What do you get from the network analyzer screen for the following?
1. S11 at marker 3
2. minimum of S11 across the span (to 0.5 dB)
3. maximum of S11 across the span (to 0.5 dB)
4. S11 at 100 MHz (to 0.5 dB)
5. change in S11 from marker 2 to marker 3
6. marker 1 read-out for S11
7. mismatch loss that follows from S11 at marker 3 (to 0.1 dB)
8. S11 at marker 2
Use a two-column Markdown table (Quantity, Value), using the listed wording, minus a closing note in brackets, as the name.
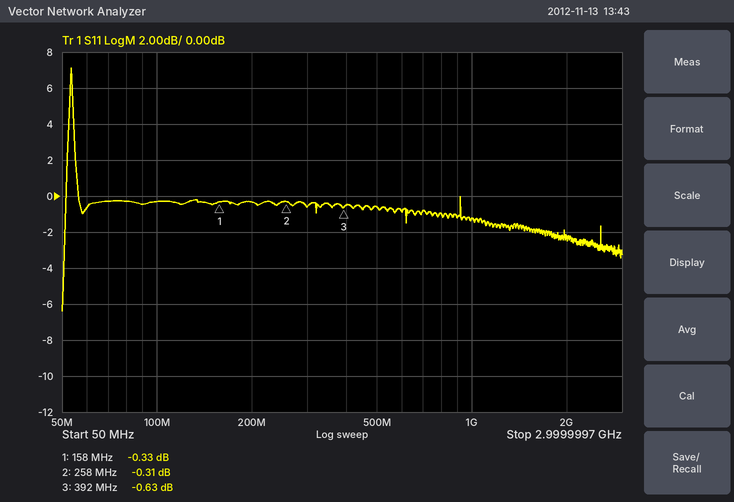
| Quantity | Value |
|---|---|
| S11 at marker 3 | -0.63 dB |
| minimum of S11 across the span | -6.5 dB |
| maximum of S11 across the span | 7.0 dB |
| S11 at 100 MHz | -0.5 dB |
| change in S11 from marker 2 to marker 3 | -0.32 dB |
| marker 1 read-out for S11 | -0.33 dB |
| mismatch loss that follows from S11 at marker 3 | 8.7 dB |
| S11 at marker 2 | -0.31 dB |
